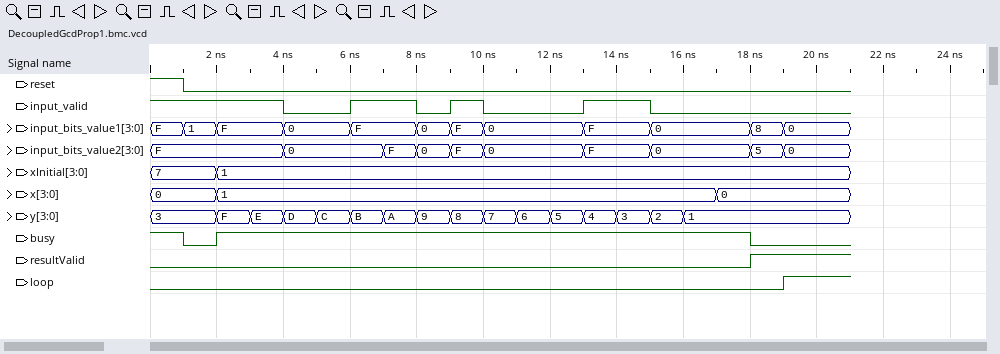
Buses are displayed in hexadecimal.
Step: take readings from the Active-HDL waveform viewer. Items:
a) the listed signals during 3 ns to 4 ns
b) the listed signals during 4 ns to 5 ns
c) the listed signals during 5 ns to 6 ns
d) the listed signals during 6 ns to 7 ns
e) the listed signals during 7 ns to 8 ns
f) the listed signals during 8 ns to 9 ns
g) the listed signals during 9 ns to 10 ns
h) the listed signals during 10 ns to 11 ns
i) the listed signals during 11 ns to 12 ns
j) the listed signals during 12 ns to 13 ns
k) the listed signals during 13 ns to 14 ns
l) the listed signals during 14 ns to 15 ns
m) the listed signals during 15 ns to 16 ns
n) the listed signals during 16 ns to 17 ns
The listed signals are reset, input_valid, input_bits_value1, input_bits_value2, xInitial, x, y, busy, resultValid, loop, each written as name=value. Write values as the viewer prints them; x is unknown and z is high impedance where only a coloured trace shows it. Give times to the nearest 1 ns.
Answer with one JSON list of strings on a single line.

["reset=0, input_valid=1, input_bits_value1=F, input_bits_value2=F, xInitial=1, x=1, y=E, busy=1, resultValid=0, loop=0", "reset=0, input_valid=0, input_bits_value1=0, input_bits_value2=0, xInitial=1, x=1, y=D, busy=1, resultValid=0, loop=0", "reset=0, input_valid=0, input_bits_value1=0, input_bits_value2=0, xInitial=1, x=1, y=C, busy=1, resultValid=0, loop=0", "reset=0, input_valid=1, input_bits_value1=F, input_bits_value2=0, xInitial=1, x=1, y=B, busy=1, resultValid=0, loop=0", "reset=0, input_valid=1, input_bits_value1=F, input_bits_value2=F, xInitial=1, x=1, y=A, busy=1, resultValid=0, loop=0", "reset=0, input_valid=0, input_bits_value1=0, input_bits_value2=0, xInitial=1, x=1, y=9, busy=1, resultValid=0, loop=0", "reset=0, input_valid=1, input_bits_value1=F, input_bits_value2=F, xInitial=1, x=1, y=8, busy=1, resultValid=0, loop=0", "reset=0, input_valid=0, input_bits_value1=0, input_bits_value2=0, xInitial=1, x=1, y=7, busy=1, resultValid=0, loop=0", "reset=0, input_valid=0, input_bits_value1=0, input_bits_value2=0, xInitial=1, x=1, y=6, busy=1, resultValid=0, loop=0", "reset=0, input_valid=0, input_bits_value1=0, input_bits_value2=0, xInitial=1, x=1, y=5, busy=1, resultValid=0, loop=0", "reset=0, input_valid=1, input_bits_value1=F, input_bits_value2=F, xInitial=1, x=1, y=4, busy=1, resultValid=0, loop=0", "reset=0, input_valid=1, input_bits_value1=F, input_bits_value2=F, xInitial=1, x=1, y=3, busy=1, resultValid=0, loop=0", "reset=0, input_valid=0, input_bits_value1=0, input_bits_value2=0, xInitial=1, x=1, y=2, busy=1, resultValid=0, loop=0", "reset=0, input_valid=0, input_bits_value1=0, input_bits_value2=0, xInitial=1, x=1, y=1, busy=1, resultValid=0, loop=0"]
